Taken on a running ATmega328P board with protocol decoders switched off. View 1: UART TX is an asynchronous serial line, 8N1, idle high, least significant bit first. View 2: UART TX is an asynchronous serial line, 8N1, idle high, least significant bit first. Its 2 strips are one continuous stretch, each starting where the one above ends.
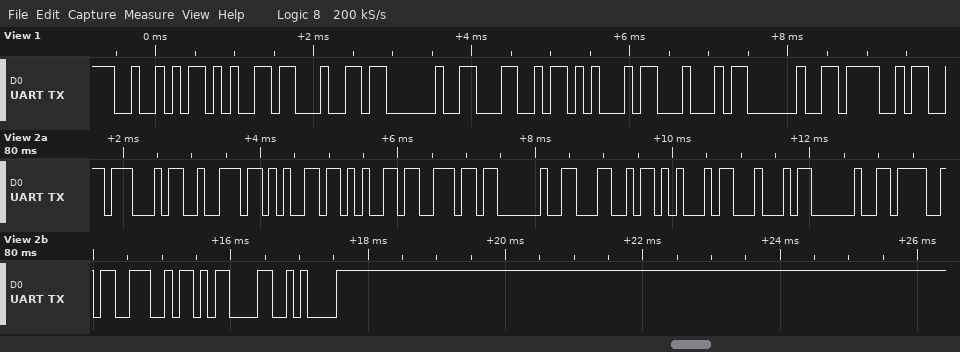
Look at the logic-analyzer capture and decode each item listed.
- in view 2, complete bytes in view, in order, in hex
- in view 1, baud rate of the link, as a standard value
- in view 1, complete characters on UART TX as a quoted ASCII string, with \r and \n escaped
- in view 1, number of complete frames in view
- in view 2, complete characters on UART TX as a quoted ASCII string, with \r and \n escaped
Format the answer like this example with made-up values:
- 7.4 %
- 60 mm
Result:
- 47 72 65 65 6E 20 4C 45 44 20 4F 4E 0D 0A
- 9600 baud
- "Red LED O"
- 9
- "Green LED ON\r\n"
